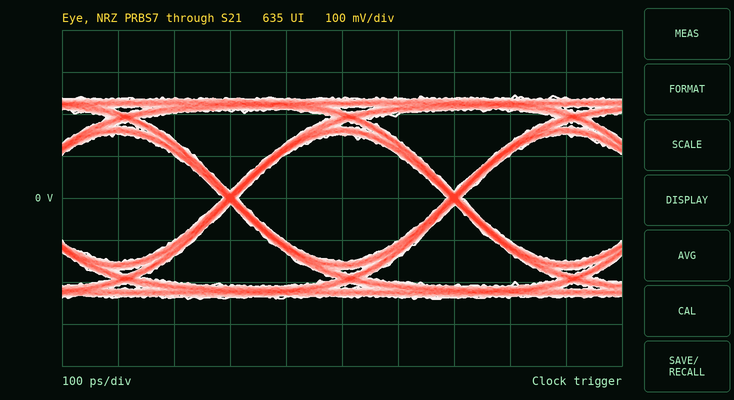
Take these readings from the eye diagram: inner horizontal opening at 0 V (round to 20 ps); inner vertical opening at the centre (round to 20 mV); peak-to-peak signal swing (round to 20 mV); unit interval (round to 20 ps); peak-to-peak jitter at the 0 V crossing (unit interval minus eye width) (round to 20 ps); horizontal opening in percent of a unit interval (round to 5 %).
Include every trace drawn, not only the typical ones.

380 ps
300 mV
480 mV
400 ps
20 ps
95 %
